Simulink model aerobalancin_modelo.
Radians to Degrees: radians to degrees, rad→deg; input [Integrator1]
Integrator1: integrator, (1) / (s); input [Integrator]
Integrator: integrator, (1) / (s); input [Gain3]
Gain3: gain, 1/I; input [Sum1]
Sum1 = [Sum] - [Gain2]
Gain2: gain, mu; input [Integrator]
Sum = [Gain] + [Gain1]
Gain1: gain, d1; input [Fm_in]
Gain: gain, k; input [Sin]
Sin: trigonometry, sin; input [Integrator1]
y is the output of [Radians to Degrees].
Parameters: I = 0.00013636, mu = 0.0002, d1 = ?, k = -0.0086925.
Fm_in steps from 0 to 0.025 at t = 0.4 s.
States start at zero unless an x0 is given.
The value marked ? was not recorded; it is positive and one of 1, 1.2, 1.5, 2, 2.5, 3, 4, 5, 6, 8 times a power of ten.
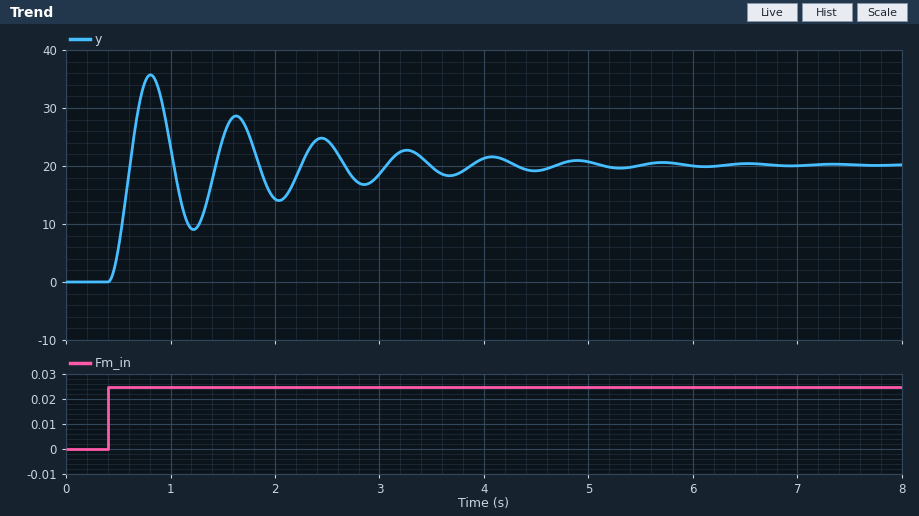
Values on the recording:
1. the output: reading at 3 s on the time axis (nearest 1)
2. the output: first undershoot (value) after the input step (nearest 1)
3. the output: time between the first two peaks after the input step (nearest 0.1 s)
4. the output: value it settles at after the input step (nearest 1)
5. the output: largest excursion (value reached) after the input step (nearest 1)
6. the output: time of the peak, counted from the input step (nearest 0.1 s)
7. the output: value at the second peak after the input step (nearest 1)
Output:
19
9
0.8 s
20
36
0.4 s
29
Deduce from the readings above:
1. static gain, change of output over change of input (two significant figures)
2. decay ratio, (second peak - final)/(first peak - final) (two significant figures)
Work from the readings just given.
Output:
800
0.56
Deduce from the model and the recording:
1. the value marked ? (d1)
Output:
0.12
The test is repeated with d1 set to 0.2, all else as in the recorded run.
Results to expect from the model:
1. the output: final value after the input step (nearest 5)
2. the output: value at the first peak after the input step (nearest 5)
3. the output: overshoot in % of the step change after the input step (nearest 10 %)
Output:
35
65
80 %
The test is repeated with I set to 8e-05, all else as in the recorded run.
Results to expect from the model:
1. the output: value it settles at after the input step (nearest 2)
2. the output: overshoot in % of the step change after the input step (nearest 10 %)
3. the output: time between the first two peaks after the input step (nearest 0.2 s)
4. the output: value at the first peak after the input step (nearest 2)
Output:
20
70 %
0.6 s
34
